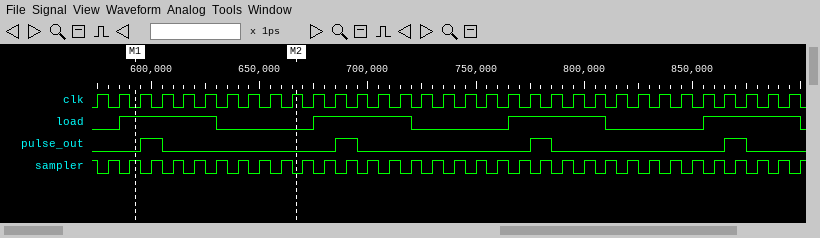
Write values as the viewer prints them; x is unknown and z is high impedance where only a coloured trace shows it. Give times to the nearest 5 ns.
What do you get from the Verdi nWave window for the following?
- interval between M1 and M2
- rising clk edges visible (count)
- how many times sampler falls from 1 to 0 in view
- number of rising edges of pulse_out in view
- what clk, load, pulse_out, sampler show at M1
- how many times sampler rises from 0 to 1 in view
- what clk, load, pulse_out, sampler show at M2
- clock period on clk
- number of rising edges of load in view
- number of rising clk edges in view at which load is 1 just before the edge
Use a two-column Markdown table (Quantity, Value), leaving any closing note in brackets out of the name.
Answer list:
| Quantity | Value |
|---|---|
| interval between M1 and M2 | 75 ns |
| rising clk edges visible | 33 |
| how many times sampler falls from 1 to 0 in view | 33 |
| number of rising edges of pulse_out in view | 4 |
| what clk, load, pulse_out, sampler show at M1 | clk=0, load=1, pulse_out=0, sampler=1 |
| how many times sampler rises from 0 to 1 in view | 33 |
| what clk, load, pulse_out, sampler show at M2 | clk=1, load=0, pulse_out=0, sampler=0 |
| clock period on clk | 10 ns |
| number of rising edges of load in view | 4 |
| number of rising clk edges in view at which load is 1 just before the edge | 16 |
